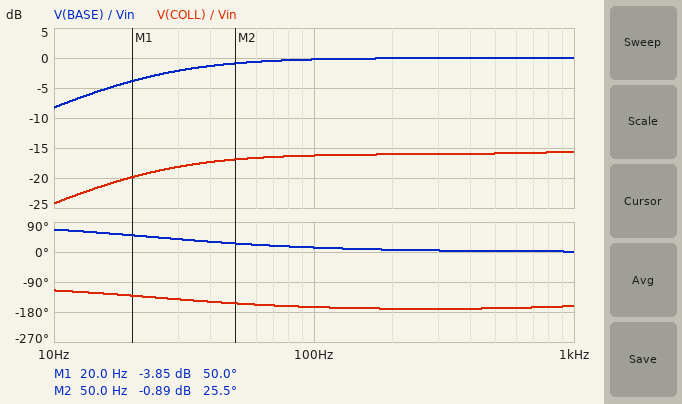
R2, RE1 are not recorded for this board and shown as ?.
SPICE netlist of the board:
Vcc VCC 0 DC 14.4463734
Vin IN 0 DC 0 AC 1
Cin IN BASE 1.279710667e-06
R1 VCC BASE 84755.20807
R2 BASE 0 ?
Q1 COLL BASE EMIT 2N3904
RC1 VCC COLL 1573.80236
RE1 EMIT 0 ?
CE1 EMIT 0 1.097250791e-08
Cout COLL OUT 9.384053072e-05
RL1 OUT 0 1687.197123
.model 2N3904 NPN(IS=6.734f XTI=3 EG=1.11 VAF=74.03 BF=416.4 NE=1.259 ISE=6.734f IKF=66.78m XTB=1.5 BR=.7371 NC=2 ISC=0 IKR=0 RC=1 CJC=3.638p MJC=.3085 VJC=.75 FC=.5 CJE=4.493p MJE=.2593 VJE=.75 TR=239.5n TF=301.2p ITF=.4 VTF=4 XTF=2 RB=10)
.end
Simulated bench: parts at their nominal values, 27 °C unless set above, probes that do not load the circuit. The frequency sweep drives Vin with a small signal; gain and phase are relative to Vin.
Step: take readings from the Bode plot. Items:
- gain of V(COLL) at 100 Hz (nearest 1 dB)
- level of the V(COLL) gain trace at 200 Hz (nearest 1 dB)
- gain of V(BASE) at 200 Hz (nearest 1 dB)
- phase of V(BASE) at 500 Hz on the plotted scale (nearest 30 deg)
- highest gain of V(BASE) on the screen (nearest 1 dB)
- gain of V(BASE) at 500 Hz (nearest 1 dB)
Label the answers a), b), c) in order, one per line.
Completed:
a) -16 dB
b) -16 dB
c) 0 dB
d) 0 deg
e) 0 dB
f) 0 dB
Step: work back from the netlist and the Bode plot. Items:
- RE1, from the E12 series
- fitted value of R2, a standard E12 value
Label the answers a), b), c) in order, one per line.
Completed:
a) 4.7 kΩ
b) 5.6 kΩ
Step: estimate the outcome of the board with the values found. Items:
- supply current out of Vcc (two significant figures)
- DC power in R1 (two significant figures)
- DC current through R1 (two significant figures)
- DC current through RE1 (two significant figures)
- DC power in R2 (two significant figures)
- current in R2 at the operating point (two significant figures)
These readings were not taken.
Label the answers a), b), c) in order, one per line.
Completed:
a) 220 µA
b) 2.2 mW
c) 160 µA
d) 64 µA
e) 140 µW
f) 160 µA
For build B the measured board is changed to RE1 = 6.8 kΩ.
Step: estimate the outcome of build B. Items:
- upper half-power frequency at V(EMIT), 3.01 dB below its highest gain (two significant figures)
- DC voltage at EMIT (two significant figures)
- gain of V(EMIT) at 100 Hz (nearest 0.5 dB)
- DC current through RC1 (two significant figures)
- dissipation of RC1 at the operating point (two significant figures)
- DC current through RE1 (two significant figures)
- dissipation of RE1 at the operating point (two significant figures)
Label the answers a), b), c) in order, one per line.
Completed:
a) 28 kHz
b) 310 mV
c) -1.0 dB
d) 45 µA
e) 3.2 µW
f) 46 µA
g) 14 µW
